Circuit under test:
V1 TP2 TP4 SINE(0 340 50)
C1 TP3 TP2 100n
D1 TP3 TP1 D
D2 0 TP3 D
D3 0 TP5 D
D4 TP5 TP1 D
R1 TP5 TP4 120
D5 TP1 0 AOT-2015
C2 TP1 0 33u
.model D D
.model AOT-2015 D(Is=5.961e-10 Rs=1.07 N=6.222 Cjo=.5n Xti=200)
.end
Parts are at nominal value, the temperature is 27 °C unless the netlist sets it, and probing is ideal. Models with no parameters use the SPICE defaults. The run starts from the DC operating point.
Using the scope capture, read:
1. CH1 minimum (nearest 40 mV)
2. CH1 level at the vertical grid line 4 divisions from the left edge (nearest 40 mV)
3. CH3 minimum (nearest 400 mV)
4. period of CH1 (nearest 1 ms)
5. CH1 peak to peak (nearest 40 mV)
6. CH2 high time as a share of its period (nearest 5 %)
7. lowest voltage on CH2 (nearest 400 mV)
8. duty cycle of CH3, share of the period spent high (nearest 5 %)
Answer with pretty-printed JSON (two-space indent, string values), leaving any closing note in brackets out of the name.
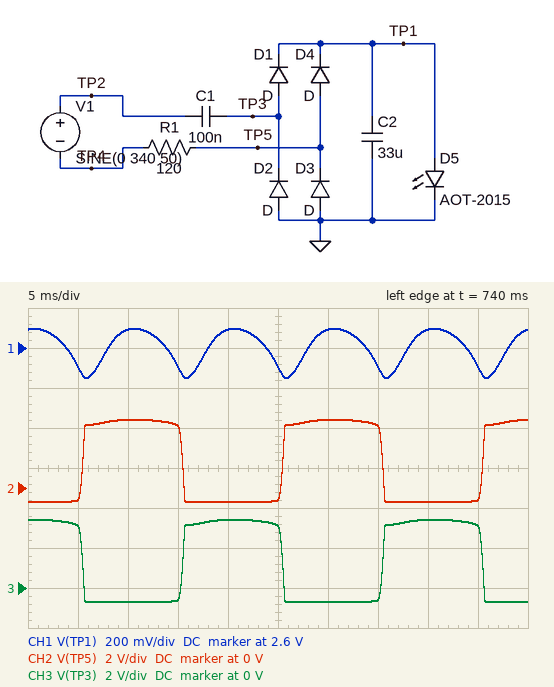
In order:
{
  "CH1 minimum": "2.44 V",
  "CH1 level at the vertical grid line 4 divisions from the left edge": "2.68 V",
  "CH3 minimum": "-800 mV",
  "period of CH1": "10 ms",
  "CH1 peak to peak": "240 mV",
  "CH2 high time as a share of its period": "50 %",
  "lowest voltage on CH2": "-800 mV",
  "duty cycle of CH3, share of the period spent high": "50 %"
}
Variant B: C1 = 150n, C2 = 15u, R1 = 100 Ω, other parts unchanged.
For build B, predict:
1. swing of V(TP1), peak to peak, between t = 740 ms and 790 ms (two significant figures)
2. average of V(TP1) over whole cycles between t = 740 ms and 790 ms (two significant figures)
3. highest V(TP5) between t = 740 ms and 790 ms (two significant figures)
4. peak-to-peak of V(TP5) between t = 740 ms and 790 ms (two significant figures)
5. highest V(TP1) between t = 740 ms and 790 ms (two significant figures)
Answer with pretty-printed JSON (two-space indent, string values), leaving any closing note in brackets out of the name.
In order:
{
  "swing of V(TP1), peak to peak, between t = 740 ms and 790 ms": "380 mV",
  "average of V(TP1) over whole cycles between t = 740 ms and 790 ms": "2.7 V",
  "highest V(TP5) between t = 740 ms and 790 ms": "3.5 V",
  "peak-to-peak of V(TP5) between t = 740 ms and 790 ms": "4.2 V",
  "highest V(TP1) between t = 740 ms and 790 ms": "2.8 V"
}
